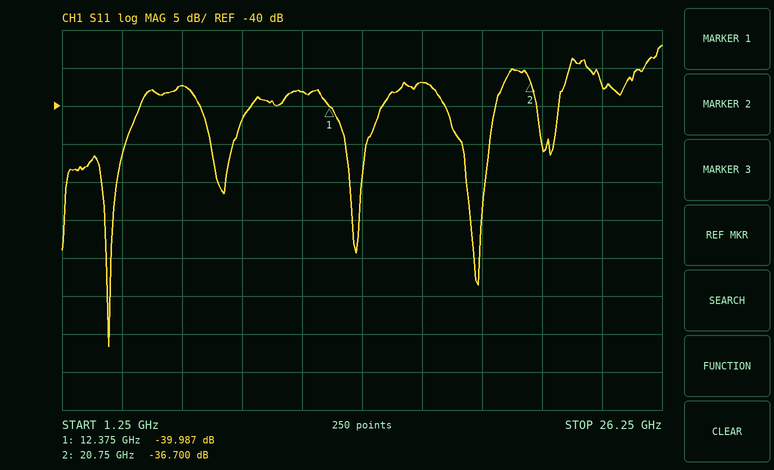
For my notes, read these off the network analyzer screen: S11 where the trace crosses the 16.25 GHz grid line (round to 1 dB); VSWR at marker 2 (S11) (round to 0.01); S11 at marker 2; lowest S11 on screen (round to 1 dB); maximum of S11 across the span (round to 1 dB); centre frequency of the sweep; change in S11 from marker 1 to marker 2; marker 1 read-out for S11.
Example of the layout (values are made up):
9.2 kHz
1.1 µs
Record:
-37 dB
1.03
-36.700 dB
-72 dB
-32 dB
13.75 GHz
3.287 dB
-39.987 dB
